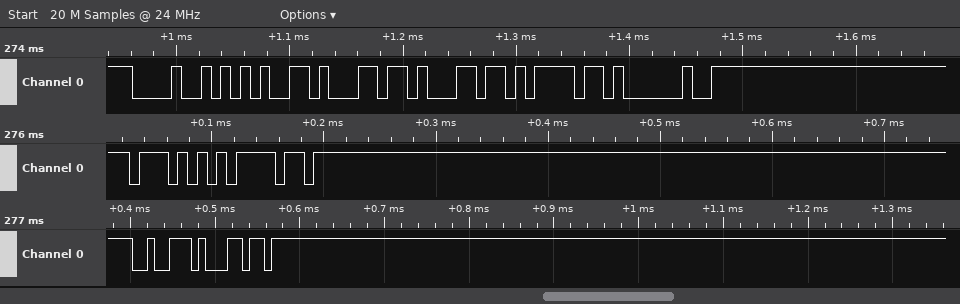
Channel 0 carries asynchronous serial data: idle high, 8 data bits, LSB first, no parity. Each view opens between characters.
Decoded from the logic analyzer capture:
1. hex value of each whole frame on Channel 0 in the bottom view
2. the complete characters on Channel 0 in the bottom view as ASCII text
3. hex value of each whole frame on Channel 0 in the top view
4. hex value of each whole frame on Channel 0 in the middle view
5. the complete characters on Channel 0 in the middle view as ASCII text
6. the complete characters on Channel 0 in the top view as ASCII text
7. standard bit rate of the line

72, 6C
"rl"
48, 65, 6C, 6C, 6F, 20
57, 6F
"Wo"
"Hello "
115200 baud
